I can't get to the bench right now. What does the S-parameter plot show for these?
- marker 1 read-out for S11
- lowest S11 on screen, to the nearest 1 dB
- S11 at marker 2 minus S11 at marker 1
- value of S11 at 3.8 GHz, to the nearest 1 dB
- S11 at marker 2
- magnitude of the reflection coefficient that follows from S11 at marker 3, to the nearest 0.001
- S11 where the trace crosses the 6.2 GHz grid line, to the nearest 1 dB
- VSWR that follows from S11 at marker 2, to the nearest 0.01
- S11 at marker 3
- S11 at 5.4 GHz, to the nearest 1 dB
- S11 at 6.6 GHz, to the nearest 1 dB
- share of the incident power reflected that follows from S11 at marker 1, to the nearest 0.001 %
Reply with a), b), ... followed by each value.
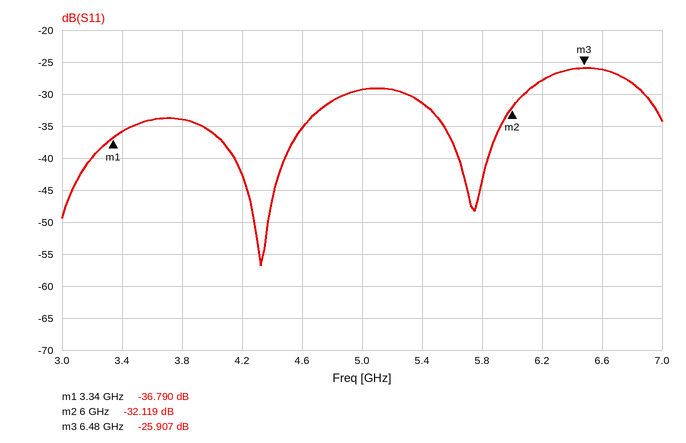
a) -36.790 dB
b) -57 dB
c) 4.671 dB
d) -34 dB
e) -32.119 dB
f) 0.051
g) -28 dB
h) 1.05
i) -25.907 dB
j) -31 dB
k) -26 dB
l) 0.021 %
